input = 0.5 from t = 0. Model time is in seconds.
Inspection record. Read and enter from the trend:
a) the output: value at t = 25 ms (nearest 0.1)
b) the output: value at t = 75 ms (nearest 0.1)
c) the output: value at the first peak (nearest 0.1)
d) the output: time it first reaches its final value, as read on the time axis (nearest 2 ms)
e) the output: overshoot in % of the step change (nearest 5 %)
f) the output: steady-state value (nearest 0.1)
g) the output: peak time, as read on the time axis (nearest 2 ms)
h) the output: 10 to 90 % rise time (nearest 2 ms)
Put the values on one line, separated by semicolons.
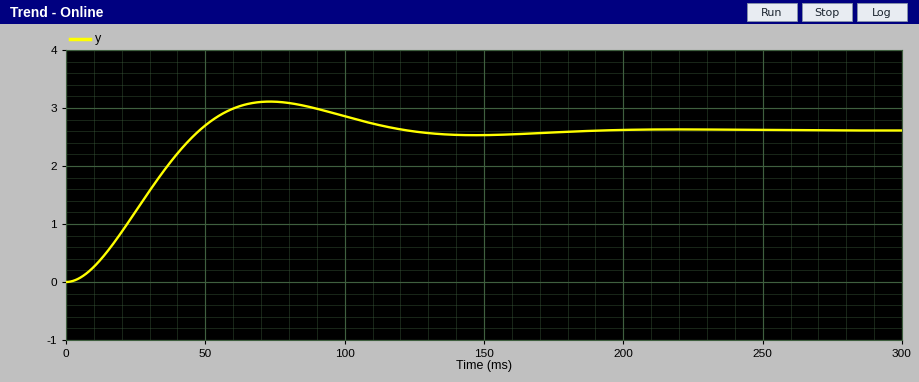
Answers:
1.2; 3.1; 3.1; 48 ms; 20 %; 2.6; 74 ms; 32 ms
